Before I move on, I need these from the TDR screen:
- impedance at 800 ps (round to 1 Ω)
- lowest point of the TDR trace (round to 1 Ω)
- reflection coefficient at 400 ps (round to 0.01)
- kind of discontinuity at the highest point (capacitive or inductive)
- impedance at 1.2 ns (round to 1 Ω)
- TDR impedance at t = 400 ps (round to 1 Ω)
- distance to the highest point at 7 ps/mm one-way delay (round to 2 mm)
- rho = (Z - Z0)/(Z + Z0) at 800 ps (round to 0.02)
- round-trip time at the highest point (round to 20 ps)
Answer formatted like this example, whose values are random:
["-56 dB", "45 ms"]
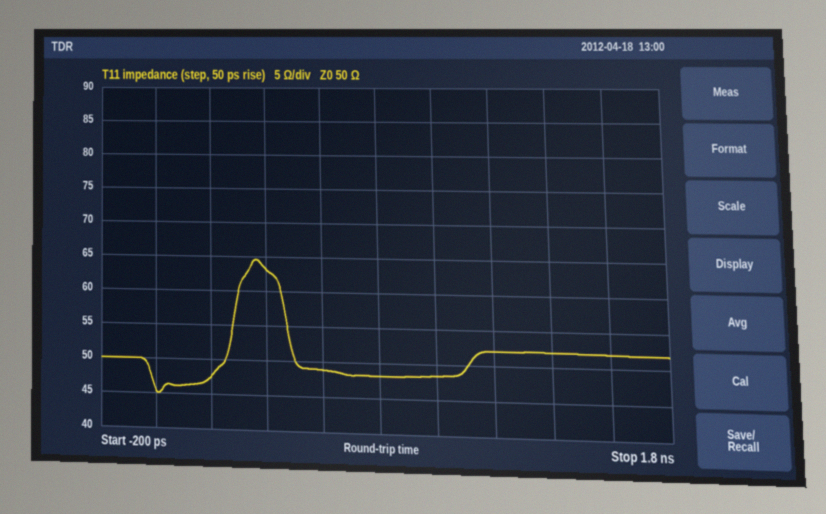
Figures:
["48 Ω", "45 Ω", "+0.12", "inductive", "52 Ω", "63 Ω", "26 mm", "-0.02", "360 ps"]
